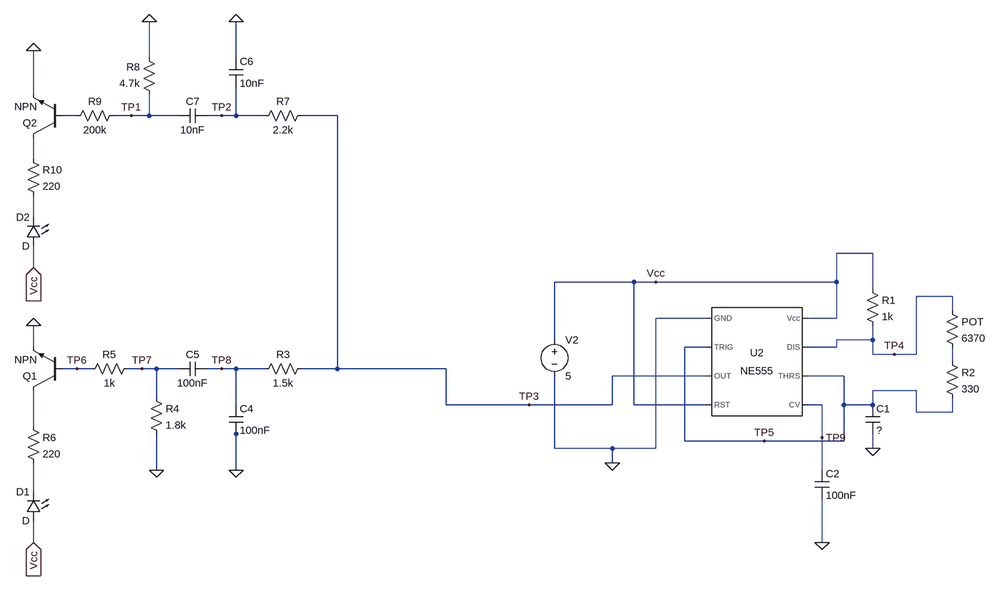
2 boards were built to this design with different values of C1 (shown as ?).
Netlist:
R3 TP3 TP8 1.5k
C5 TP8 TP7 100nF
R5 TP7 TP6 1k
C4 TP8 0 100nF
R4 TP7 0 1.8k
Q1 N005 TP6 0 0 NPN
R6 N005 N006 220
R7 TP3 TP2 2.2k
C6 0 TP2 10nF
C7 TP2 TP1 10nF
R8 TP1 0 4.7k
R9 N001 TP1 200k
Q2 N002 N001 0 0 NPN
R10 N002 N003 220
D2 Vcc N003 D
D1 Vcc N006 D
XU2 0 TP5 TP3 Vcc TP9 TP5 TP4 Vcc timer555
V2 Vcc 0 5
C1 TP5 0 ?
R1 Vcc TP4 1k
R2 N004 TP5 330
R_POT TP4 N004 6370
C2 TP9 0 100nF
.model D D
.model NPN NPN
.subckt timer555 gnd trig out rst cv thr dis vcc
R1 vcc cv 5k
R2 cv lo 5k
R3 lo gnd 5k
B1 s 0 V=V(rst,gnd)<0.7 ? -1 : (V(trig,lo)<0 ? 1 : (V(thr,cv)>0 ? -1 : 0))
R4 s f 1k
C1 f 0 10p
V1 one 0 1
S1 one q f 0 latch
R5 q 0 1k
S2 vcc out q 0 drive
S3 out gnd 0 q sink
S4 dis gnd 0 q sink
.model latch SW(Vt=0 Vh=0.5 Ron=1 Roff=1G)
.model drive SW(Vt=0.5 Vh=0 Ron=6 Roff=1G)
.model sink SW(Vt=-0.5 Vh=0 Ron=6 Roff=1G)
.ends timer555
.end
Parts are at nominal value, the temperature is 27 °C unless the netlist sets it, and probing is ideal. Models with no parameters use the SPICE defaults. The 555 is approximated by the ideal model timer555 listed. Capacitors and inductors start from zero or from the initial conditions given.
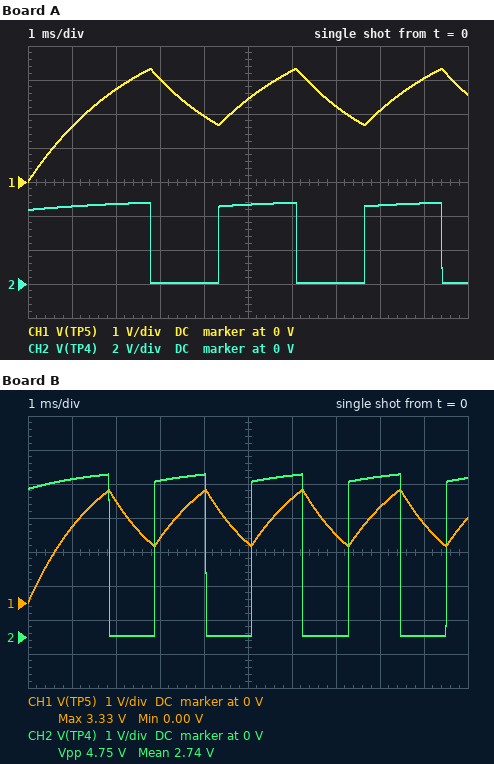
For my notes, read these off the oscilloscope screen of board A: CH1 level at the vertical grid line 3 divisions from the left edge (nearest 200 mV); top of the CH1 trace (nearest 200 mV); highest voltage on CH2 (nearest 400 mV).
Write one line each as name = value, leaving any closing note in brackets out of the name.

CH1 level at the vertical grid line 3 divisions from the left edge = 3.0 V
top of the CH1 trace = 3.4 V
highest voltage on CH2 = 4.8 V
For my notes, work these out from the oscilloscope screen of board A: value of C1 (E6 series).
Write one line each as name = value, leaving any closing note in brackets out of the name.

value of C1 = 330 nF
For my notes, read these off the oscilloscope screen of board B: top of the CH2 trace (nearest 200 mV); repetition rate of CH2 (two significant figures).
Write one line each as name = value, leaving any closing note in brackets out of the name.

top of the CH2 trace = 4.8 V
repetition rate of CH2 = 450 Hz
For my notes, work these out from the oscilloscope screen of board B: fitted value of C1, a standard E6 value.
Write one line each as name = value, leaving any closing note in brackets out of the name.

fitted value of C1, a standard E6 value = 220 nF
